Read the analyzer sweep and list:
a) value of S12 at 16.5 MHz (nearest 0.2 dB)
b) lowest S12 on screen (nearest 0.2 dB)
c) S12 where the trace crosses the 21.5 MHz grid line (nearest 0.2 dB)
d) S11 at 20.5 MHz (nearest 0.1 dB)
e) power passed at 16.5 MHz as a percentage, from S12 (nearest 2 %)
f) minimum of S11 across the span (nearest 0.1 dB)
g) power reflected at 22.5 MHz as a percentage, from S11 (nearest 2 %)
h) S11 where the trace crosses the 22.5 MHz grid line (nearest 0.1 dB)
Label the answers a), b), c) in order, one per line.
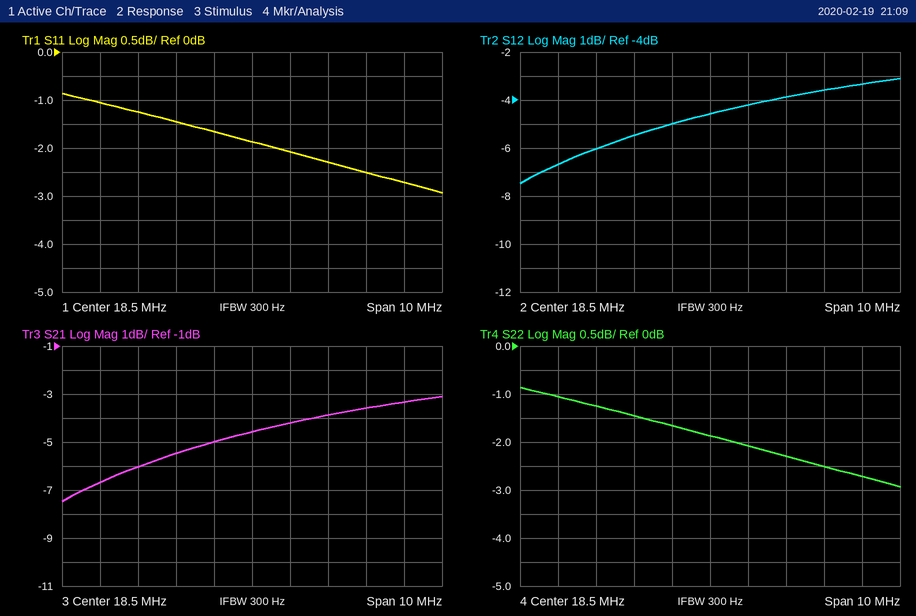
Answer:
a) -5.4 dB
b) -7.4 dB
c) -3.6 dB
d) -2.3 dB
e) 28 %
f) -2.9 dB
g) 54 %
h) -2.7 dB
